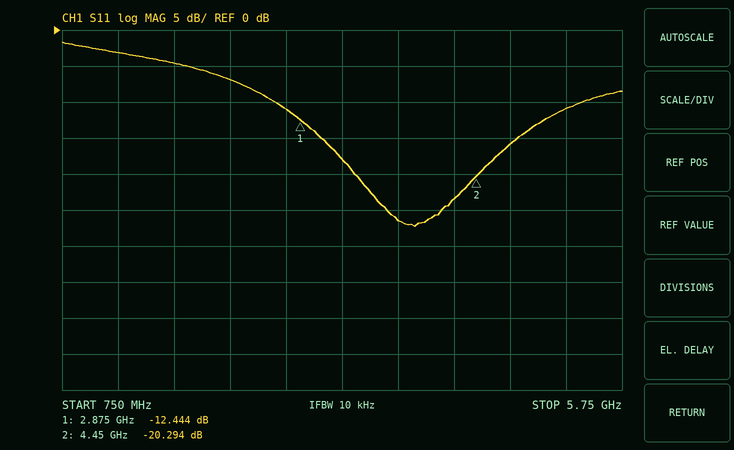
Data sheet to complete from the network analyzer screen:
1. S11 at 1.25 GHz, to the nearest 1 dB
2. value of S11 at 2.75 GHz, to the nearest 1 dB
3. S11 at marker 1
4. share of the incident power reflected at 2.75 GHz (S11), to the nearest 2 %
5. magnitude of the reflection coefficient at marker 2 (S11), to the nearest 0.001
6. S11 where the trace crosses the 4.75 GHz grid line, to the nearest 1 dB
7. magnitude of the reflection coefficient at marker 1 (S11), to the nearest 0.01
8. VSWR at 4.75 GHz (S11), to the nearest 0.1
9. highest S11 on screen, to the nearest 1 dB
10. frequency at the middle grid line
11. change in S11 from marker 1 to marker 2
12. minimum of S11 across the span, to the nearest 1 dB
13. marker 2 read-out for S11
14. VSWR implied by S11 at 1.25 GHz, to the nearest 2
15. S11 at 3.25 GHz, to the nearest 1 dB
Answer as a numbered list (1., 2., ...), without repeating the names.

1. -3 dB
2. -11 dB
3. -12.444 dB
4. 8 %
5. 0.097
6. -16 dB
7. 0.24
8. 1.4
9. -2 dB
10. 3.25 GHz
11. -7.850 dB
12. -27 dB
13. -20.294 dB
14. 6
15. -18 dB
